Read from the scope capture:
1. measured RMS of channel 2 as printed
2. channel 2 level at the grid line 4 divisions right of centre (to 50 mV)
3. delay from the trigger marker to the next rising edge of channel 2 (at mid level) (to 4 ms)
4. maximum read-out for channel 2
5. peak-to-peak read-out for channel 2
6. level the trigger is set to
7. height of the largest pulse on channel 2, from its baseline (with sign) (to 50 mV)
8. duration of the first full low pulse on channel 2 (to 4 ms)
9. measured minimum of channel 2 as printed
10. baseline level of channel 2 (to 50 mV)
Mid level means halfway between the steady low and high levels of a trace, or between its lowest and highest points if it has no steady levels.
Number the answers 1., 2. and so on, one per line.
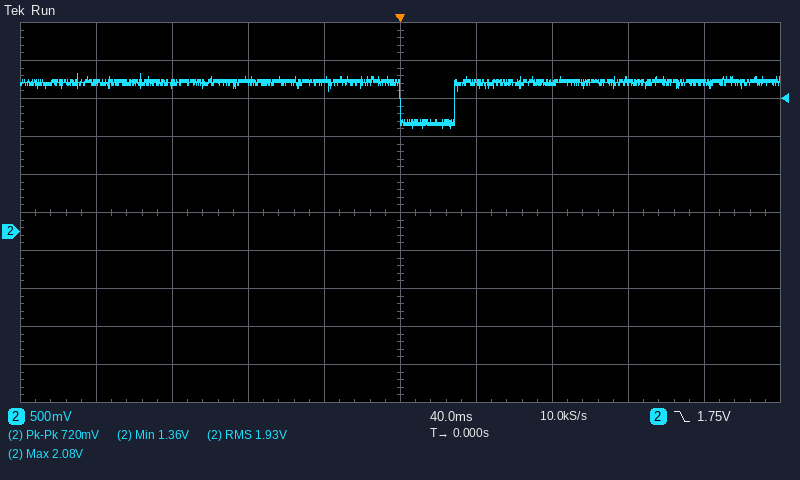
1. 1.93 V
2. 1.95 V
3. 28 ms
4. 2.08 V
5. 720 mV
6. 1.75 V
7. -600 mV
8. 28 ms
9. 1.36 V
10. 1.95 V
